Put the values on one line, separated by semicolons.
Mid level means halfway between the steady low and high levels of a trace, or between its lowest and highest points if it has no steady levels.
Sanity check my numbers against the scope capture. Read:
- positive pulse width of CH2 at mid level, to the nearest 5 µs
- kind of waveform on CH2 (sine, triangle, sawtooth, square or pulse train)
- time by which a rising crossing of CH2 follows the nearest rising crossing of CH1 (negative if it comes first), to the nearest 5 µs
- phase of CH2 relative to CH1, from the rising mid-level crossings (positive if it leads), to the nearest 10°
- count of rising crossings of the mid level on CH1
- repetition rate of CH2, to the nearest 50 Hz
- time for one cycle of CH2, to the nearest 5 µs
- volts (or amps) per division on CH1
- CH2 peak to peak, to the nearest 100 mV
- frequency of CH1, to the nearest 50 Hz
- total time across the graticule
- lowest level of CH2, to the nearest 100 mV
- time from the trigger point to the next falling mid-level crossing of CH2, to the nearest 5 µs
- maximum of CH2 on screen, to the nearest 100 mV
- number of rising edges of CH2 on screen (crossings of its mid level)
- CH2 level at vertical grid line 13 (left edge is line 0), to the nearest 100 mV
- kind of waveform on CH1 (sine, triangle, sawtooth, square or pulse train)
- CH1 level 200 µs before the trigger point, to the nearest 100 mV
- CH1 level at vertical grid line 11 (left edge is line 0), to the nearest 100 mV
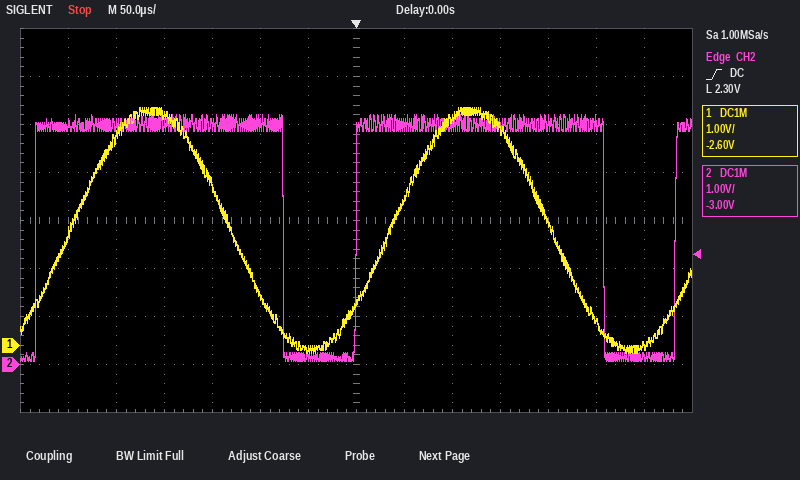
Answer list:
260 µs; pulse train; -35 µs; +40°; 2; 3.00 kHz; 335 µs; 1 V; 5.1 V; 3.00 kHz; 700 µs; 100 mV; 260 µs; 5.2 V; 3; 200 mV; sine; 4.8 V; 2.6 V
